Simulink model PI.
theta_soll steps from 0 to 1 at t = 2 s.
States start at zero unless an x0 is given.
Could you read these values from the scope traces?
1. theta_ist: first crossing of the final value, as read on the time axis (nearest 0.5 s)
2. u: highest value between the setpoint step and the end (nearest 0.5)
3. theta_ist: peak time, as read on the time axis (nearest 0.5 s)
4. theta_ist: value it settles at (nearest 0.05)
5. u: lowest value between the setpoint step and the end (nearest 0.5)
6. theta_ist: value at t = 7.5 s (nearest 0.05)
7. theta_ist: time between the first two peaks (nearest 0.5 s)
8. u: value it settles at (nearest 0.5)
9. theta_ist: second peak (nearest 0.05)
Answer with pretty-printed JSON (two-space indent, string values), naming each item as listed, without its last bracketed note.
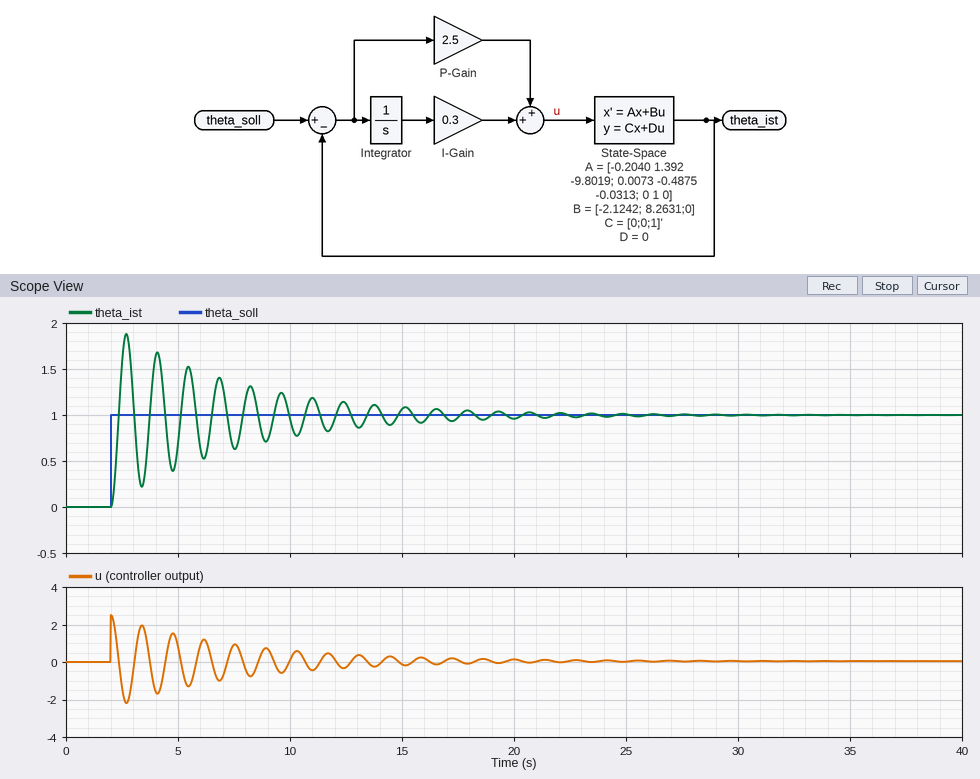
{
  "theta_ist: first crossing of the final value, as read on the time axis": "2.5 s",
  "u: highest value between the setpoint step and the end": "2.5",
  "theta_ist: peak time, as read on the time axis": "2.5 s",
  "theta_ist: value it settles at": "1.00",
  "u: lowest value between the setpoint step and the end": "-2.0",
  "theta_ist: value at t = 7.5 s": "0.65",
  "theta_ist: time between the first two peaks": "1.5 s",
  "u: value it settles at": "0.0",
  "theta_ist: second peak": "1.70"
}
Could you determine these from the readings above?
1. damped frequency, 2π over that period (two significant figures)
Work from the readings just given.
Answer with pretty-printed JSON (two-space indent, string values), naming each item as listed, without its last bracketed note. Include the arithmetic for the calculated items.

{
  "damped frequency, 2π over that period": "2π / 1.5 = 4.2 rad/s"
}
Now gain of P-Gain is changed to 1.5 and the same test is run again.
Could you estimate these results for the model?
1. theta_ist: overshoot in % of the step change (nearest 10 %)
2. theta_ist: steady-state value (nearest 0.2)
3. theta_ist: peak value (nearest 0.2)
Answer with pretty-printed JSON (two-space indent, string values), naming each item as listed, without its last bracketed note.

{
  "theta_ist: overshoot in % of the step change": "90 %",
  "theta_ist: steady-state value": "1.0",
  "theta_ist: peak value": "1.8"
}
